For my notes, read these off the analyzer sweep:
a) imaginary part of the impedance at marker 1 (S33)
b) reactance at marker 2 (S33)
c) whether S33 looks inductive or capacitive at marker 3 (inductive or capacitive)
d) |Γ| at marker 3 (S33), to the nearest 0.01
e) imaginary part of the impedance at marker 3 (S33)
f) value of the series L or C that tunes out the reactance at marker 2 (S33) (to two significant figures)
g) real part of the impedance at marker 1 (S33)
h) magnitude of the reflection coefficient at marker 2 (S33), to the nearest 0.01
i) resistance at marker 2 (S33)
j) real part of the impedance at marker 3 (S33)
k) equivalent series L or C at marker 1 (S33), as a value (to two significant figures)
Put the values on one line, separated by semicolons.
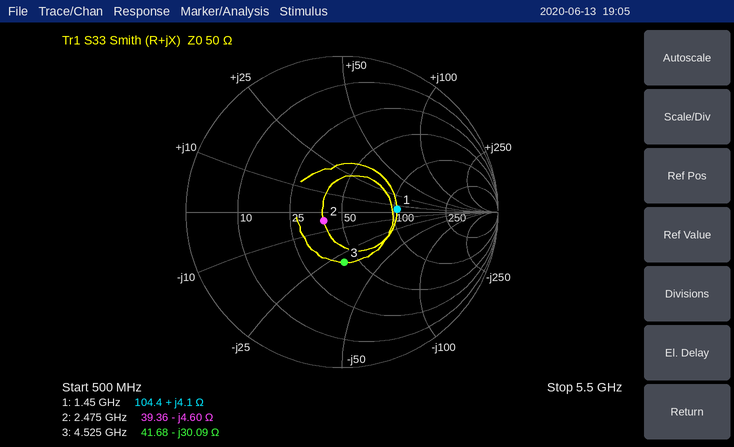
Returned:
+4.1 Ω; -4.60 Ω; capacitive; 0.32; -30.09 Ω; 300 pH; 104.4 Ω; 0.13; 39.36 Ω; 41.68 Ω; 450 pH
